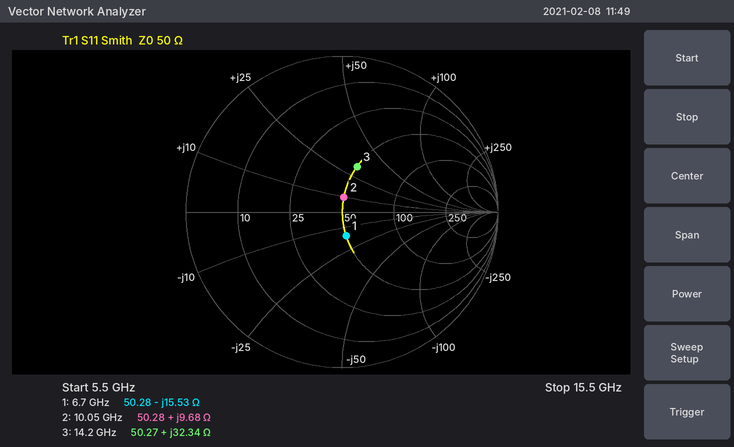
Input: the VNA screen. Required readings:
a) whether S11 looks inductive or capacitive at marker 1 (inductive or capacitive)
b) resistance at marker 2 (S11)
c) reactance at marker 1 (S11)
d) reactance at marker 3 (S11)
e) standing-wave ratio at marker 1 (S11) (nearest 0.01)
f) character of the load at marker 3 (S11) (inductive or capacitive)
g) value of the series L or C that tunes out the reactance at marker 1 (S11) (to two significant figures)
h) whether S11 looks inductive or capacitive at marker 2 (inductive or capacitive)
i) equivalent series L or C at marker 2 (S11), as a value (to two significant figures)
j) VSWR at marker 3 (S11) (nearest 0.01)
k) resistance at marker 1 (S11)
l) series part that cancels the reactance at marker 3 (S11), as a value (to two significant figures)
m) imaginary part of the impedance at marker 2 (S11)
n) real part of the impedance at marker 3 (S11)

capacitive
50.28 Ω
-15.53 Ω
+32.34 Ω
1.36
inductive
370 pH
inductive
150 pH
1.89
50.28 Ω
350 fF
+9.68 Ω
50.27 Ω
